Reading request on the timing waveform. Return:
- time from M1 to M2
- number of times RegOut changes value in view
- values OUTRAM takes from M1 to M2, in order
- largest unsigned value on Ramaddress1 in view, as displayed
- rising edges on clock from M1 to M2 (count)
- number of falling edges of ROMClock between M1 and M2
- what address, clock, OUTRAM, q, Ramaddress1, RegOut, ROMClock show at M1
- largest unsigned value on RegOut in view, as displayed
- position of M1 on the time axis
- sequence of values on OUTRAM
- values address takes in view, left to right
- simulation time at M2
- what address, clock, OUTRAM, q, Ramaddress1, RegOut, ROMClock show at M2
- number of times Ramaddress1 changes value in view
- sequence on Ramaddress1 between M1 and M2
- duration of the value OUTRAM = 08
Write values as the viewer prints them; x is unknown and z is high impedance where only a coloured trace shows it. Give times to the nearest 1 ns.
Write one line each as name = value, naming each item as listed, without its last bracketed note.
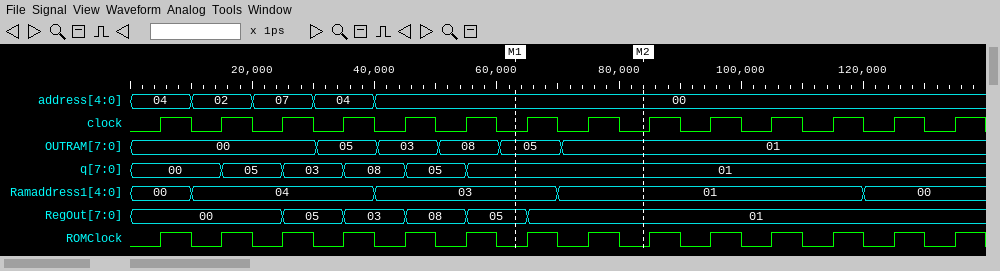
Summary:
time from M1 to M2 = 21 ns
number of times RegOut changes value in view = 5
values OUTRAM takes from M1 to M2, in order = 05, 01
largest unsigned value on Ramaddress1 in view, as displayed = 04
rising edges on clock from M1 to M2 = 2
number of falling edges of ROMClock between M1 and M2 = 2
what address, clock, OUTRAM, q, Ramaddress1, RegOut, ROMClock show at M1 = address=00, clock=0, OUTRAM=05, q=01, Ramaddress1=03, RegOut=05, ROMClock=0
largest unsigned value on RegOut in view, as displayed = 08
position of M1 on the time axis = 63 ns
sequence of values on OUTRAM = 00, 05, 03, 08, 05, 01
values address takes in view, left to right = 04, 02, 07, 04, 00
simulation time at M2 = 84 ns
what address, clock, OUTRAM, q, Ramaddress1, RegOut, ROMClock show at M2 = address=00, clock=0, OUTRAM=01, q=01, Ramaddress1=01, RegOut=01, ROMClock=0
number of times Ramaddress1 changes value in view = 4
sequence on Ramaddress1 between M1 and M2 = 03, 01
duration of the value OUTRAM = 08 = 10 ns
